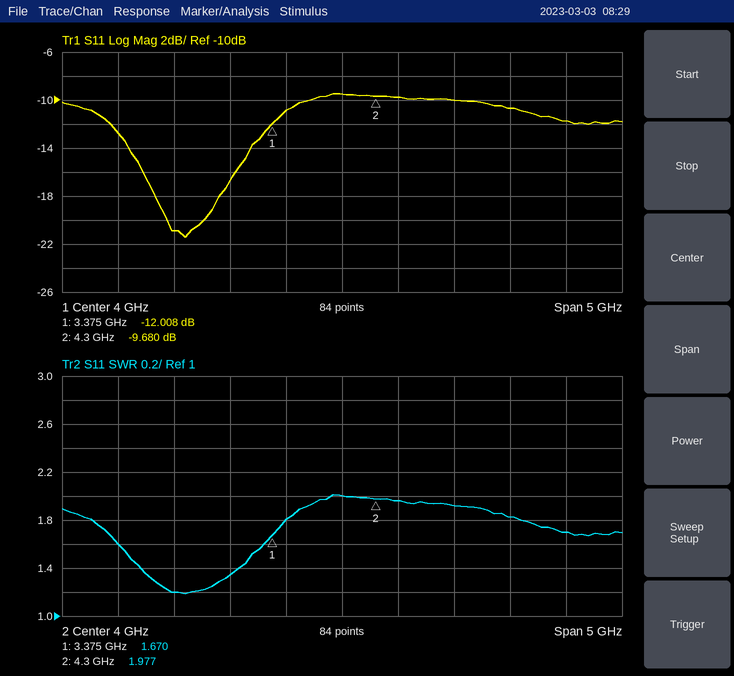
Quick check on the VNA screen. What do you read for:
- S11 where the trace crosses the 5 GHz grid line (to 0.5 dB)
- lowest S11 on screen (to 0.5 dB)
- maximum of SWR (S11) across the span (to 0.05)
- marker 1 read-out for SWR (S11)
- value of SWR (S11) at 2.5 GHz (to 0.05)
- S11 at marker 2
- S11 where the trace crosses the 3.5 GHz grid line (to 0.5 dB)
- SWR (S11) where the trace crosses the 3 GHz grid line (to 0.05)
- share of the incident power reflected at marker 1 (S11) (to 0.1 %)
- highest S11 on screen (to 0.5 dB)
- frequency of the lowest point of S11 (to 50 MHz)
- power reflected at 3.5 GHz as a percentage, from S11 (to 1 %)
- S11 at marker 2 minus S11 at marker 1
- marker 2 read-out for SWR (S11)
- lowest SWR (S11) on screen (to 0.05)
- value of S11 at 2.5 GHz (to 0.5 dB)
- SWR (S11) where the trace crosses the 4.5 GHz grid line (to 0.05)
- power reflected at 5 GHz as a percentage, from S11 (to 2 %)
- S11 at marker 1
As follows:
-10.0 dB
-21.5 dB
2.00
1.670
1.20
-9.680 dB
-11.0 dB
1.35
6.3 %
-9.5 dB
2.60 GHz
8 %
2.328 dB
1.977
1.20
-21.0 dB
1.95
10 %
-12.008 dB
